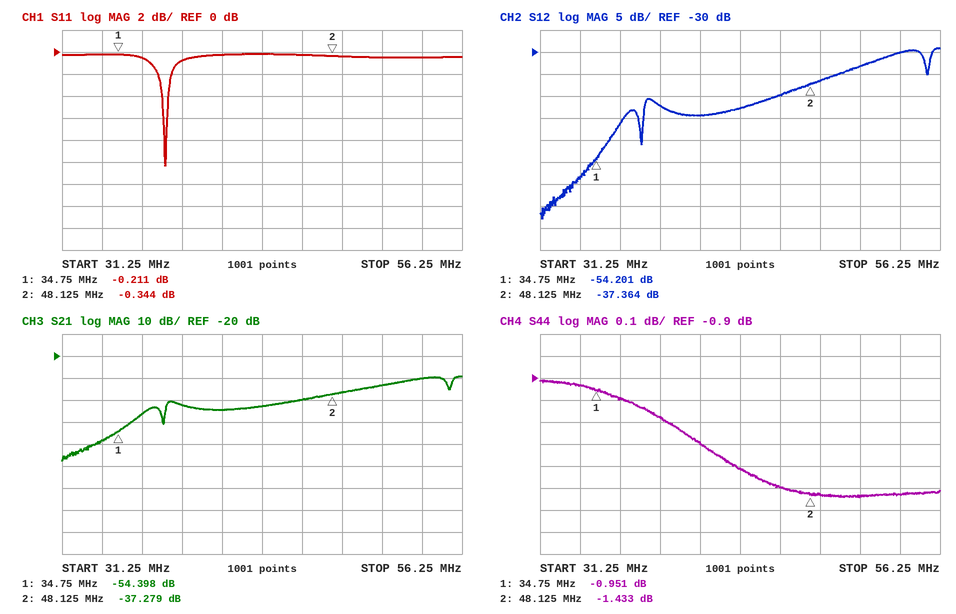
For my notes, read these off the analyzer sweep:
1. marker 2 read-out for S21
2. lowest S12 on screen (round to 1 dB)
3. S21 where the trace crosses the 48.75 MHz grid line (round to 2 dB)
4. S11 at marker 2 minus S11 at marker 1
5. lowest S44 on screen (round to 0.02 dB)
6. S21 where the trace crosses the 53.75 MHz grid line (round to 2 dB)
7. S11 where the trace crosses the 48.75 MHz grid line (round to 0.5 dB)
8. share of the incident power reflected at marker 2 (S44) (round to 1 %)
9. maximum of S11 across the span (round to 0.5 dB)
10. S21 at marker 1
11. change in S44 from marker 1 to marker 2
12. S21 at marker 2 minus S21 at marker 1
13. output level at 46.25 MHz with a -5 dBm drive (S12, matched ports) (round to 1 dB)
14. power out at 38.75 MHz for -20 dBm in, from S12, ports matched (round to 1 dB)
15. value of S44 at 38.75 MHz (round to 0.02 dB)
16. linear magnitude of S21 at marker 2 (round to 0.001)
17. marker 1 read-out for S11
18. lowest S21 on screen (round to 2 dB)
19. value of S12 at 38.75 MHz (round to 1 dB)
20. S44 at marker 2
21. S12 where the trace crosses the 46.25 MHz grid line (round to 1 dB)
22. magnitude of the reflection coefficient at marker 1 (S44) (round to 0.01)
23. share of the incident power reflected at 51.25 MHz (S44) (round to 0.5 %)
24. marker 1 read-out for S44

-37.279 dB
-68 dB
-36 dB
-0.133 dB
-1.44 dB
-30 dB
-0.5 dB
72 %
0.0 dB
-54.398 dB
-0.482 dB
17.119 dB
-45 dBm
-62 dBm
-1.08 dB
0.014
-0.211 dB
-68 dB
-42 dB
-1.433 dB
-40 dB
0.90
72.0 %
-0.951 dB
